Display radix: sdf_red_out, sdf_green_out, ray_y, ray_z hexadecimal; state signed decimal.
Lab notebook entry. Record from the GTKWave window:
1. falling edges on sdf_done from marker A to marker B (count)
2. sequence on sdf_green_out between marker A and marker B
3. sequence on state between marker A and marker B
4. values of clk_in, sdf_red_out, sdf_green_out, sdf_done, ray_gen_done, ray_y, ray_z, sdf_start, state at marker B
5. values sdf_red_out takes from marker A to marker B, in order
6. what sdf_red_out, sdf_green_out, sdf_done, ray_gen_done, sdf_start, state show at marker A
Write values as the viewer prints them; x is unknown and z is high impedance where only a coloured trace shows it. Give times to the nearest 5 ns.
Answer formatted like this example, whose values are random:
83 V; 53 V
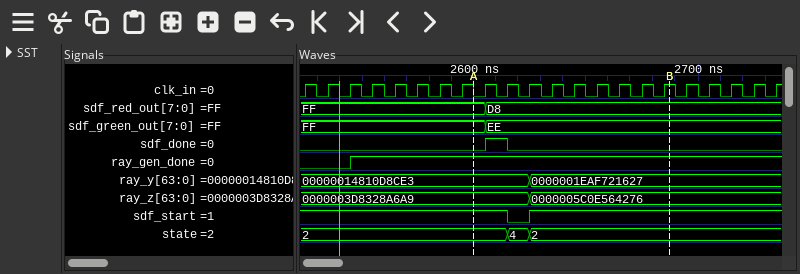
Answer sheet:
1; FF, EE; 2, 4, 2; clk_in=1, sdf_red_out=D8, sdf_green_out=EE, sdf_done=0, ray_gen_done=1, ray_y=0000001EAF721627, ray_z=0000005C0E564276, sdf_start=1, state=2; FF, D8; sdf_red_out=FF, sdf_green_out=FF, sdf_done=0, ray_gen_done=1, sdf_start=1, state=2
